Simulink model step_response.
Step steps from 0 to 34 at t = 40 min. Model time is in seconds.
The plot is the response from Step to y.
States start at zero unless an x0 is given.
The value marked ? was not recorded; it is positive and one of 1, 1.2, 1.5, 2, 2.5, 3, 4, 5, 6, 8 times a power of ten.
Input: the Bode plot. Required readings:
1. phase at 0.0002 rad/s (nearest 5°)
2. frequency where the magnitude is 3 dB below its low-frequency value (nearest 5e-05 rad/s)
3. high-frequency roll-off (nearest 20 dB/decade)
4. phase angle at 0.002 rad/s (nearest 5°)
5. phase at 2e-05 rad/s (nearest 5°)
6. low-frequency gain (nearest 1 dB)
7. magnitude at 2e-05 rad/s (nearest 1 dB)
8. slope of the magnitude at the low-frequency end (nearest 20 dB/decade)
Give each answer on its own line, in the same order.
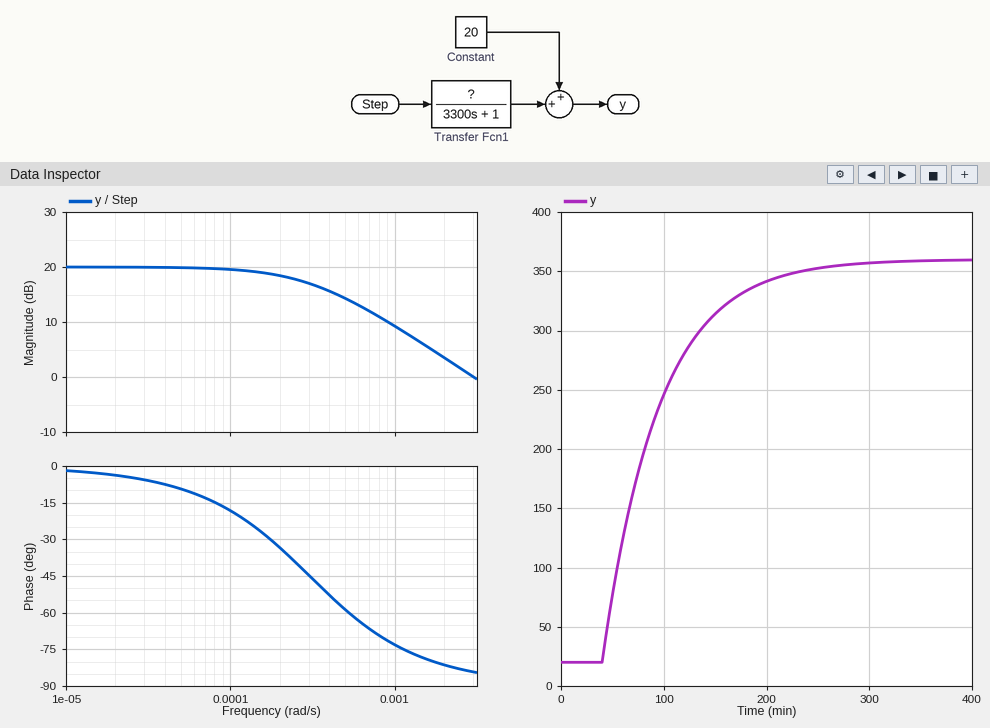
-35°
0.00030 rad/s
-20 dB/decade
-80°
-5°
20 dB
20 dB
0 dB/decade
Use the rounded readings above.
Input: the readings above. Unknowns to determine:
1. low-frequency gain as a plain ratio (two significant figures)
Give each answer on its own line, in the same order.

10
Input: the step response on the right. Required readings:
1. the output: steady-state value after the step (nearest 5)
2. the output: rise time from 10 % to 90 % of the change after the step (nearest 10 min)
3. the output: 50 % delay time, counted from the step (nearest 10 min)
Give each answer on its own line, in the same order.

360
120 min
40 min
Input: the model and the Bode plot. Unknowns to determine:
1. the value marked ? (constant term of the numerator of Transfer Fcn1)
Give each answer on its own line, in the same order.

10
